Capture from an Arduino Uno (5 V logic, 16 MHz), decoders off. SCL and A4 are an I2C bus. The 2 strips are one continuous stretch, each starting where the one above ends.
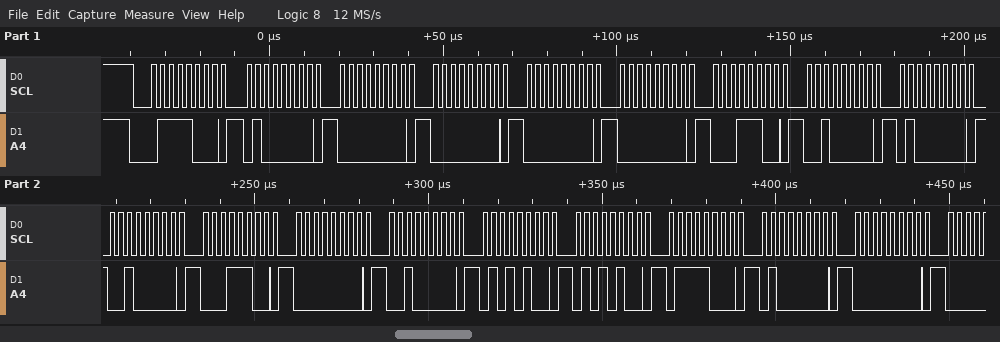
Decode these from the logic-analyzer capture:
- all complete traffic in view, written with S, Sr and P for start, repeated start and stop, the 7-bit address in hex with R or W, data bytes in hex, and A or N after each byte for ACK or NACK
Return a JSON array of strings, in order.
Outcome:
["S 3CW A 40 A 00 A 00 A 00 A 00 A 1C A 20 A 40 A 20 A 1C A 00 A 20 A 54 A 54 A 78 A 40 A 00 A"]
